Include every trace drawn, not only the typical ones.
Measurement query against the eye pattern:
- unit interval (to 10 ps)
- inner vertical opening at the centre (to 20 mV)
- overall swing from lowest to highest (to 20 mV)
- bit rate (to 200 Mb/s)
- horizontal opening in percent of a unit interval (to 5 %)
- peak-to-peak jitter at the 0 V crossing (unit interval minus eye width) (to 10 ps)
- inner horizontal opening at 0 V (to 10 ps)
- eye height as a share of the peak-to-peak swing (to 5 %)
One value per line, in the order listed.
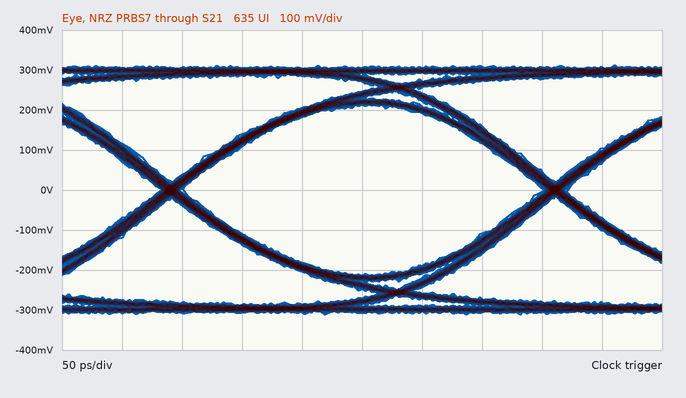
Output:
320 ps
420 mV
620 mV
3.2 Gb/s
95 %
20 ps
300 ps
70 %
